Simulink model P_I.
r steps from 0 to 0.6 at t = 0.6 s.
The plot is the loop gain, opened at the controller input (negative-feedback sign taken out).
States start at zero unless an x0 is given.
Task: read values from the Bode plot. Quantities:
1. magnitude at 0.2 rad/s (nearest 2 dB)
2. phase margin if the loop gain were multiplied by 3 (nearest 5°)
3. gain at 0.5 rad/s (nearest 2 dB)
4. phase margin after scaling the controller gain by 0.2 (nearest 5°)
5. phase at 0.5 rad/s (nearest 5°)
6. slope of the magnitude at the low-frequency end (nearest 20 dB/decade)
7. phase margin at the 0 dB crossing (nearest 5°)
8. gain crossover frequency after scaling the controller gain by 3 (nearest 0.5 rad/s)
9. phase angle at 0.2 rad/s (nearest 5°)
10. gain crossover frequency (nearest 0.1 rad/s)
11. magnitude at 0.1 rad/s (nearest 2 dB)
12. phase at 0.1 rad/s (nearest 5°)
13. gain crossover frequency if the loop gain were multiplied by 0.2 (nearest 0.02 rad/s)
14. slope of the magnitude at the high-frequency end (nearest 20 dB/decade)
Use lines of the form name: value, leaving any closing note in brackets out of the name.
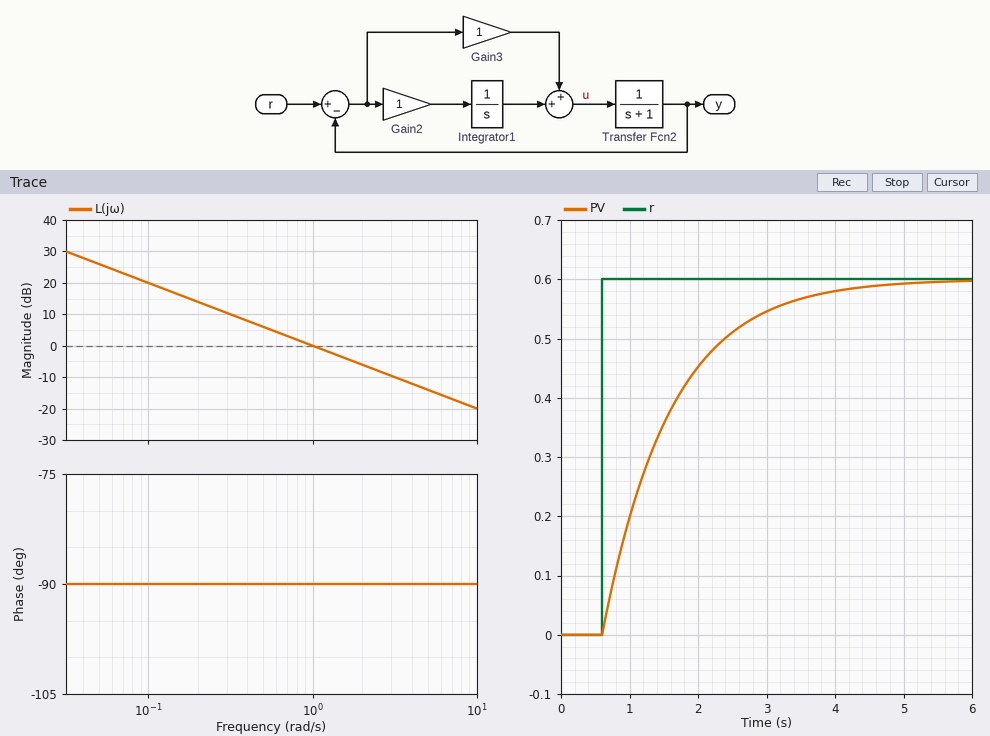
magnitude at 0.2 rad/s: 14 dB
phase margin if the loop gain were multiplied by 3: 90°
gain at 0.5 rad/s: 6 dB
phase margin after scaling the controller gain by 0.2: 90°
phase at 0.5 rad/s: -90°
slope of the magnitude at the low-frequency end: -20 dB/decade
phase margin at the 0 dB crossing: 90°
gain crossover frequency after scaling the controller gain by 3: 3.0 rad/s
phase angle at 0.2 rad/s: -90°
gain crossover frequency: 1.0 rad/s
magnitude at 0.1 rad/s: 20 dB
phase at 0.1 rad/s: -90°
gain crossover frequency if the loop gain were multiplied by 0.2: 0.20 rad/s
slope of the magnitude at the high-frequency end: -20 dB/decade
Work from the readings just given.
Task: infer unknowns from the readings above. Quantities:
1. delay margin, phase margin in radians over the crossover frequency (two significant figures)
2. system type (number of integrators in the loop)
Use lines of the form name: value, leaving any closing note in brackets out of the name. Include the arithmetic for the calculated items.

delay margin, phase margin in radians over the crossover frequency: 90 × π / 180 / 1 = 1.6 s
system type: 1
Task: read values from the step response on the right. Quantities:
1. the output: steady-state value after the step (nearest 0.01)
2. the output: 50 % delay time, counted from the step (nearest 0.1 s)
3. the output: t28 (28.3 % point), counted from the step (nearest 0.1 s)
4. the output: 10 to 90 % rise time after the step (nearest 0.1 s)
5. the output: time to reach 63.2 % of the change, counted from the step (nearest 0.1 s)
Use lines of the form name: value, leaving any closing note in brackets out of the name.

the output: steady-state value after the step: 0.60
the output: 50 % delay time, counted from the step: 0.7 s
the output: t28 (28.3 % point), counted from the step: 0.3 s
the output: 10 to 90 % rise time after the step: 2.2 s
the output: time to reach 63.2 % of the change, counted from the step: 1.0 s
